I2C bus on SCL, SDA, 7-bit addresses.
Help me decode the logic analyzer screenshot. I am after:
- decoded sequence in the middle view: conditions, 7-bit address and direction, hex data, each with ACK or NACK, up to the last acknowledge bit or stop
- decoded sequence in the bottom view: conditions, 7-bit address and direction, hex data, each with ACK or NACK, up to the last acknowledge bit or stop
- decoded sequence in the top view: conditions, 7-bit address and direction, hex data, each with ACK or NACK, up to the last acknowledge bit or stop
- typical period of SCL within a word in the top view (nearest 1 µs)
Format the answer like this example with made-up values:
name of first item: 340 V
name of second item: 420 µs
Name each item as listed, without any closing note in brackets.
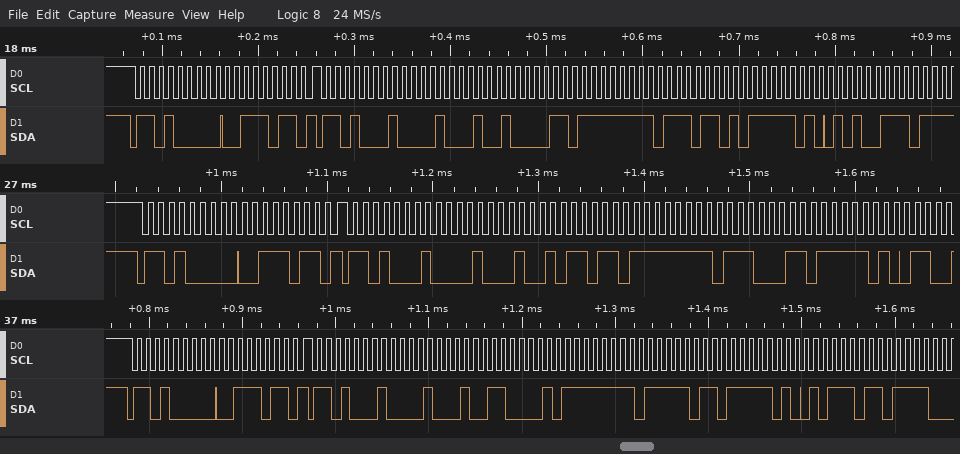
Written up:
decoded sequence in the middle view: conditions, 7-bit address and direction, hex data, each with ACK or NACK, up to the last acknowledge bit or stop: start, address 68 write ACK, 3B ACK, repeated start, address 68 read ACK, 11 ACK, 5B ACK, FF ACK, E3 ACK, FA ACK
decoded sequence in the bottom view: conditions, 7-bit address and direction, hex data, each with ACK or NACK, up to the last acknowledge bit or stop: start, address 68 write ACK, 3B ACK, repeated start, address 68 read ACK, 11 ACK, 61 ACK, FF ACK, FB ACK, FA ACK, BB ACK
decoded sequence in the top view: conditions, 7-bit address and direction, hex data, each with ACK or NACK, up to the last acknowledge bit or stop: start, address 68 write ACK, 3B ACK, repeated start, address 68 read ACK, 11 ACK, 43 ACK, FF ACK, ED ACK, FA ACK, A7 ACK
typical period of SCL within a word in the top view: 10 µs
